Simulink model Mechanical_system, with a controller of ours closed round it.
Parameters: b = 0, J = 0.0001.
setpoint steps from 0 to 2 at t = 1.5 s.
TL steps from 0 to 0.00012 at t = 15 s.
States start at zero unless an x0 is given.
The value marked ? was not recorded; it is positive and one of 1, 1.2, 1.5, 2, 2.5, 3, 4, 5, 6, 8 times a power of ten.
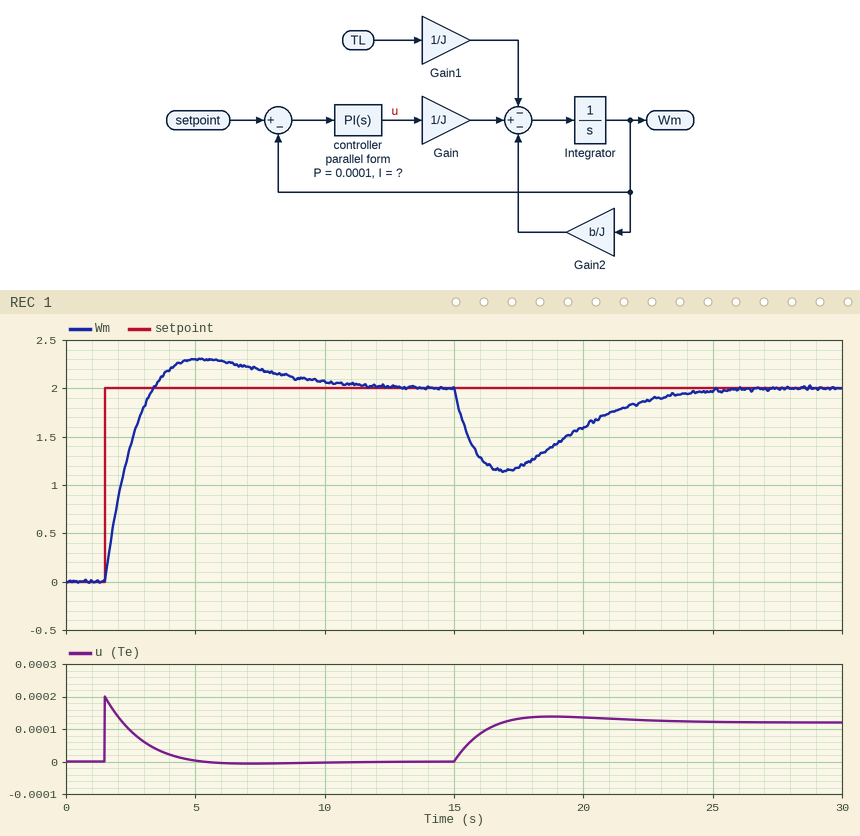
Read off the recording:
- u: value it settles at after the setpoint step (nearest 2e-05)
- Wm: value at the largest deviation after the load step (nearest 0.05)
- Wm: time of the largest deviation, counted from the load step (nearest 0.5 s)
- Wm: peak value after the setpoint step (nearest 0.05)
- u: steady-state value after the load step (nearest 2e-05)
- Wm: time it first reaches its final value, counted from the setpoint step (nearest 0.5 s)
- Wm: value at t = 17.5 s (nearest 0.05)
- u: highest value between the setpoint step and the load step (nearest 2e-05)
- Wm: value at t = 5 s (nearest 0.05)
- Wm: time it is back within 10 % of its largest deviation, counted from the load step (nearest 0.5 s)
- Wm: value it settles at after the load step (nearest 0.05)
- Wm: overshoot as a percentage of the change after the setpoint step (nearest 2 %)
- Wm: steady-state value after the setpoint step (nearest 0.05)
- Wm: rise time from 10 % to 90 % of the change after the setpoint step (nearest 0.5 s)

0.00000
1.15
2.0 s
2.30
0.00012
2.0 s
1.20
0.00020
2.30
8.0 s
2.00
16 %
2.00
1.5 s
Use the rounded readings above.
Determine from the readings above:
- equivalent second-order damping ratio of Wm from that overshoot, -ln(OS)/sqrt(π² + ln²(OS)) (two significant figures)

0.50
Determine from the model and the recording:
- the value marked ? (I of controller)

3e-05
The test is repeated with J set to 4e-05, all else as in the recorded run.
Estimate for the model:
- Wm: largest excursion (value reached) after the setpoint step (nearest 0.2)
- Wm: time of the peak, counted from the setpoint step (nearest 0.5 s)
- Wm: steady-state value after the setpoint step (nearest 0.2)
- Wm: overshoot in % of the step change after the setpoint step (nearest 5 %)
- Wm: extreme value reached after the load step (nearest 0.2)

2.2
2.0 s
2.0
10 %
1.0
